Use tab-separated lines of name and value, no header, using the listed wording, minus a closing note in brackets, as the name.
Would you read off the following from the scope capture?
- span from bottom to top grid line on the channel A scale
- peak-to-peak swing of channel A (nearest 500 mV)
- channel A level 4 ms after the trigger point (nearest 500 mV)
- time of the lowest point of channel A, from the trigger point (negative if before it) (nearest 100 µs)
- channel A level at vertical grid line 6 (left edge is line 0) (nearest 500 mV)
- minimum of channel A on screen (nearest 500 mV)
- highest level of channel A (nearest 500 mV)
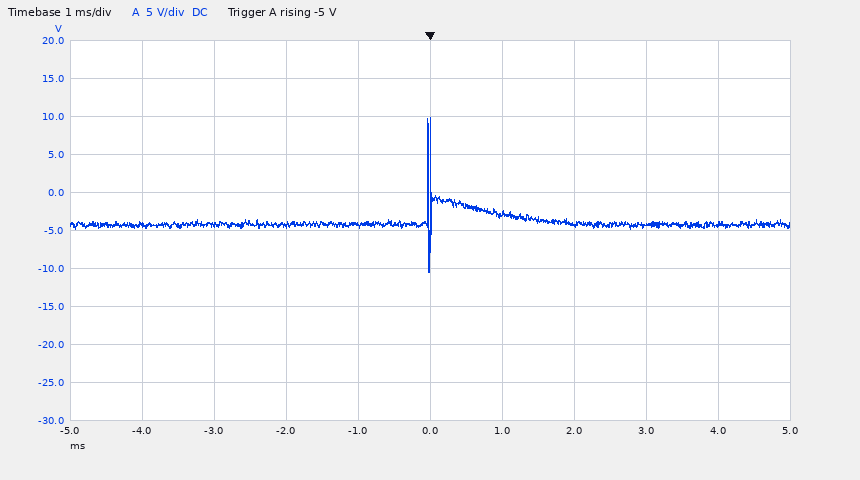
span from bottom to top grid line on the channel A scale	50 V
peak-to-peak swing of channel A	20.5 V
channel A level 4 ms after the trigger point	-4.0 V
time of the lowest point of channel A, from the trigger point (negative if before it)	0.0 ms
channel A level at vertical grid line 6 (left edge is line 0)	-3.0 V
minimum of channel A on screen	-10.5 V
highest level of channel A	10.0 V
